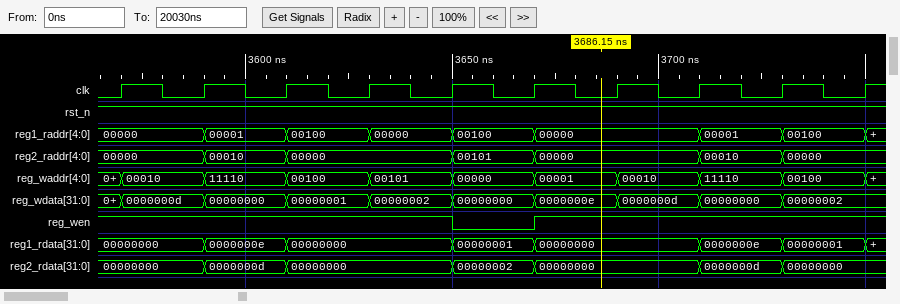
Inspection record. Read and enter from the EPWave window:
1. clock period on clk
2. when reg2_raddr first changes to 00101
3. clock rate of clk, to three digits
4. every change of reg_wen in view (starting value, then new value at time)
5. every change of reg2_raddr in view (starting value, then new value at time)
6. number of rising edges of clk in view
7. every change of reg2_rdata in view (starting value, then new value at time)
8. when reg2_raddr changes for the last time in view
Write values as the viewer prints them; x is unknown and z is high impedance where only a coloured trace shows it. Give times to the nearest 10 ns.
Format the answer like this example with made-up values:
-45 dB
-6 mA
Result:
20 ns
3650 ns
50.0 MHz
1, 0 at 3650 ns, 1 at 3670 ns
00000, 00010 at 3590 ns, 00000 at 3610 ns, 00101 at 3650 ns, 00000 at 3670 ns, 00010 at 3710 ns, 00000 at 3730 ns
10
00000000, 0000000d at 3590 ns, 00000000 at 3610 ns, 00000002 at 3650 ns, 00000000 at 3670 ns, 0000000d at 3710 ns, 00000000 at 3730 ns
3730 ns
